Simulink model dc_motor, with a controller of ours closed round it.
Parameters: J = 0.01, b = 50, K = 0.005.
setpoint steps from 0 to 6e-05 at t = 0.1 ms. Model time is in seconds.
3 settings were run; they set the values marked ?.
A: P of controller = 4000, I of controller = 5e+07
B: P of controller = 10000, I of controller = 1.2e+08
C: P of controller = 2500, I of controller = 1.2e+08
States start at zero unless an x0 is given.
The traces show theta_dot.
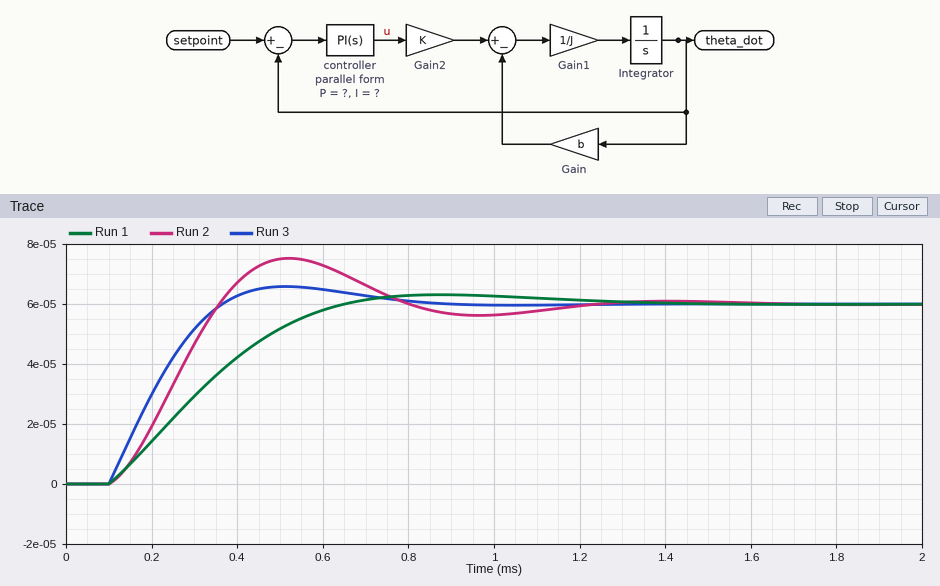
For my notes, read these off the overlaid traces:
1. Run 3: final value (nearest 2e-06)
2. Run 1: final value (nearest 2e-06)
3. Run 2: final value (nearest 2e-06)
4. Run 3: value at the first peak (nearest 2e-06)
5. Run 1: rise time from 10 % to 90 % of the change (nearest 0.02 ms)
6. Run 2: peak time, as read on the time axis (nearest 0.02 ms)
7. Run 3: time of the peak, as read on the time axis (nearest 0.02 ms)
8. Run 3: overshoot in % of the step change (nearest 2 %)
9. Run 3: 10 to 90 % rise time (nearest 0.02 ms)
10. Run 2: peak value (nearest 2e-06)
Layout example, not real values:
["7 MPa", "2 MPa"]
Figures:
["0.000060", "0.000060", "0.000060", "0.000066", "0.38 ms", "0.52 ms", "0.52 ms", "10 %", "0.20 ms", "0.000076"]
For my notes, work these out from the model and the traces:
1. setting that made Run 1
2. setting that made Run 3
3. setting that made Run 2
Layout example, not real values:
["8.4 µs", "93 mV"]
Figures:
["A", "B", "C"]
